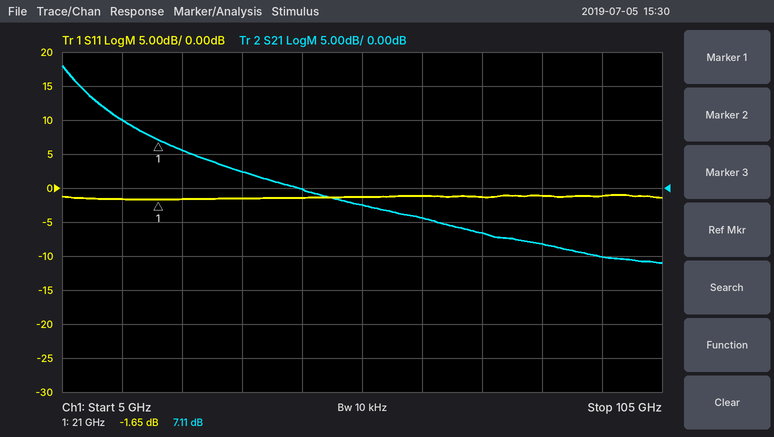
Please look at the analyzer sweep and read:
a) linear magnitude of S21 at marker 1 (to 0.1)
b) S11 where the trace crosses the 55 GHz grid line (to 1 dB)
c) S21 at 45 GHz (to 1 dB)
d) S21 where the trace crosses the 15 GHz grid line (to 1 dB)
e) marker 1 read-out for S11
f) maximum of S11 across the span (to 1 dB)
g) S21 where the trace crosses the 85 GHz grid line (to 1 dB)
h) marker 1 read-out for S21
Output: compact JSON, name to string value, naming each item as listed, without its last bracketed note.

{"linear magnitude of S21 at marker 1": "2.3", "S11 where the trace crosses the 55 GHz grid line": "-1 dB", "S21 at 45 GHz": "0 dB", "S21 where the trace crosses the 15 GHz grid line": "10 dB", "marker 1 read-out for S11": "-1.65 dB", "maximum of S11 across the span": "-1 dB", "S21 where the trace crosses the 85 GHz grid line": "-8 dB", "marker 1 read-out for S21": "7.11 dB"}
